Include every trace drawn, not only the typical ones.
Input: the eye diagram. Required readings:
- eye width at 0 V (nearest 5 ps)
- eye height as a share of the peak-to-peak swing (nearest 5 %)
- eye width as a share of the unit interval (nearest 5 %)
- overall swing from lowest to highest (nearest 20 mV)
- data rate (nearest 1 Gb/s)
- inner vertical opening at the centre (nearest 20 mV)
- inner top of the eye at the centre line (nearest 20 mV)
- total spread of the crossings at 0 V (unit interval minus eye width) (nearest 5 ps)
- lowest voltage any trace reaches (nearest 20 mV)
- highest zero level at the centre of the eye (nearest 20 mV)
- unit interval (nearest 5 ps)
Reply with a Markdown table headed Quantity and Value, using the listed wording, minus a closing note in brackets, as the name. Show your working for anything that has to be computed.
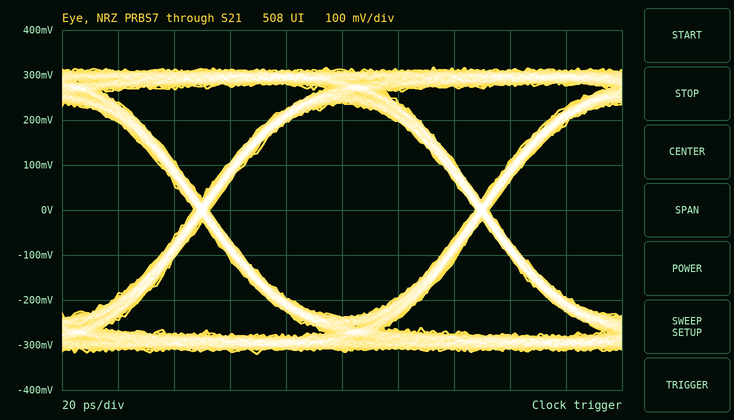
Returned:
| Quantity | Value |
|---|---|
| eye width at 0 V | 95 ps |
| eye height as a share of the peak-to-peak swing | 480 mV / 640 mV ≈ 75 % |
| eye width as a share of the unit interval | 95 ps / 100 ps ≈ 95 % |
| overall swing from lowest to highest | 640 mV |
| data rate | 10 Gb/s |
| inner vertical opening at the centre | 480 mV |
| inner top of the eye at the centre line | 240 mV |
| total spread of the crossings at 0 V (unit interval minus eye width) | 5 ps |
| lowest voltage any trace reaches | -320 mV |
| highest zero level at the centre of the eye | -240 mV |
| unit interval | 100 ps |
